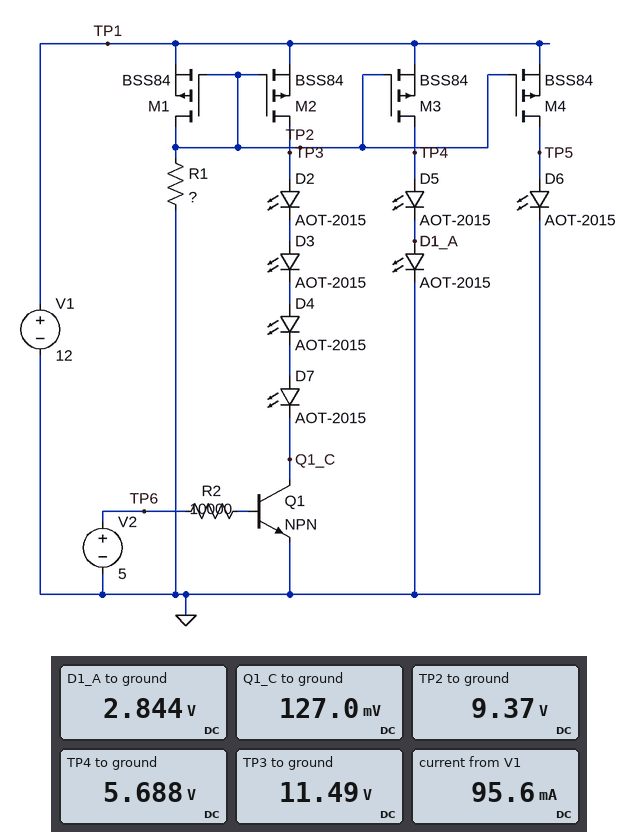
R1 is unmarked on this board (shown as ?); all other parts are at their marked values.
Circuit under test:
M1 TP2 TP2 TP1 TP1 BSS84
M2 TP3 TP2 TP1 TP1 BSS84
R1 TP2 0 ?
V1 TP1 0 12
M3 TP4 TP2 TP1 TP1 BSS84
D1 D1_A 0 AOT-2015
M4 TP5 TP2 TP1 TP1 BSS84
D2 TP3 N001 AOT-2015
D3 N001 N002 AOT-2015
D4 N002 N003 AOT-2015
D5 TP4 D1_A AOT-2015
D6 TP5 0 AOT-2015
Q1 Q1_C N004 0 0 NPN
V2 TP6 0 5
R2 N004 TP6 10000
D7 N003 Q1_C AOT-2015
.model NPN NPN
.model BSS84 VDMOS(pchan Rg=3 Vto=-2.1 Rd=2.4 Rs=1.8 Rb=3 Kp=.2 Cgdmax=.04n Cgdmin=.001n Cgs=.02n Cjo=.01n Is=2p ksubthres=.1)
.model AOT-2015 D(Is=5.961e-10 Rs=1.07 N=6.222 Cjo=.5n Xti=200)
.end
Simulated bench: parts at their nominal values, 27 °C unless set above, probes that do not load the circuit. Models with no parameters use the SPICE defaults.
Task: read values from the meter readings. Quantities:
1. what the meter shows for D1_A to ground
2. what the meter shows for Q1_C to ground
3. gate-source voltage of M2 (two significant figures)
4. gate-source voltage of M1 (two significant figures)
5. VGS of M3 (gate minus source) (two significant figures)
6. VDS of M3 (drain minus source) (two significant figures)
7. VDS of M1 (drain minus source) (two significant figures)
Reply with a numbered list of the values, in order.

1. 2.844 V
2. 127.0 mV
3. -2.6 V
4. -2.6 V
5. -2.6 V
6. -6.3 V
7. -2.6 V
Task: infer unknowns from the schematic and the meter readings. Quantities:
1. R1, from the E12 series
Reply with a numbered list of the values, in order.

1. 390 Ω
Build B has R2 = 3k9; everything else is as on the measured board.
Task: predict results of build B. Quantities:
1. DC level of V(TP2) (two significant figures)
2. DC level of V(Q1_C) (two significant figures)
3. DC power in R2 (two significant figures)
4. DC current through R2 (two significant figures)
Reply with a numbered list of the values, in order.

1. 9.4 V
2. 89 mV
3. 4.4 mW
4. 1.1 mA
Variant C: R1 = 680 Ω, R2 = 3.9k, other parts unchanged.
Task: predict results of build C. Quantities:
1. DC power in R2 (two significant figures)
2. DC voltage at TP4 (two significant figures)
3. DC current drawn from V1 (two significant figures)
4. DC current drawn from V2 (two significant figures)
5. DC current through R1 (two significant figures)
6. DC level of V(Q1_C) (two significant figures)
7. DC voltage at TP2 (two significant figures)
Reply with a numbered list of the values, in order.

1. 4.4 mW
2. 5.5 V
3. 56 mA
4. 1.1 mA
5. 14 mA
6. 74 mV
7. 9.5 V
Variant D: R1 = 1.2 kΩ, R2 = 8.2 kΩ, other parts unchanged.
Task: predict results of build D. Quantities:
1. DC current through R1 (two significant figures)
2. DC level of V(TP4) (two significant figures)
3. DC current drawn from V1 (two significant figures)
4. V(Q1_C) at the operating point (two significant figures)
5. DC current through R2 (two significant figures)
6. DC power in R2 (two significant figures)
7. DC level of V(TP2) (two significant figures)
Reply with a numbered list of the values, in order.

1. 8.0 mA
2. 5.3 V
3. 32 mA
4. 79 mV
5. 510 µA
6. 2.1 mW
7. 9.6 V
